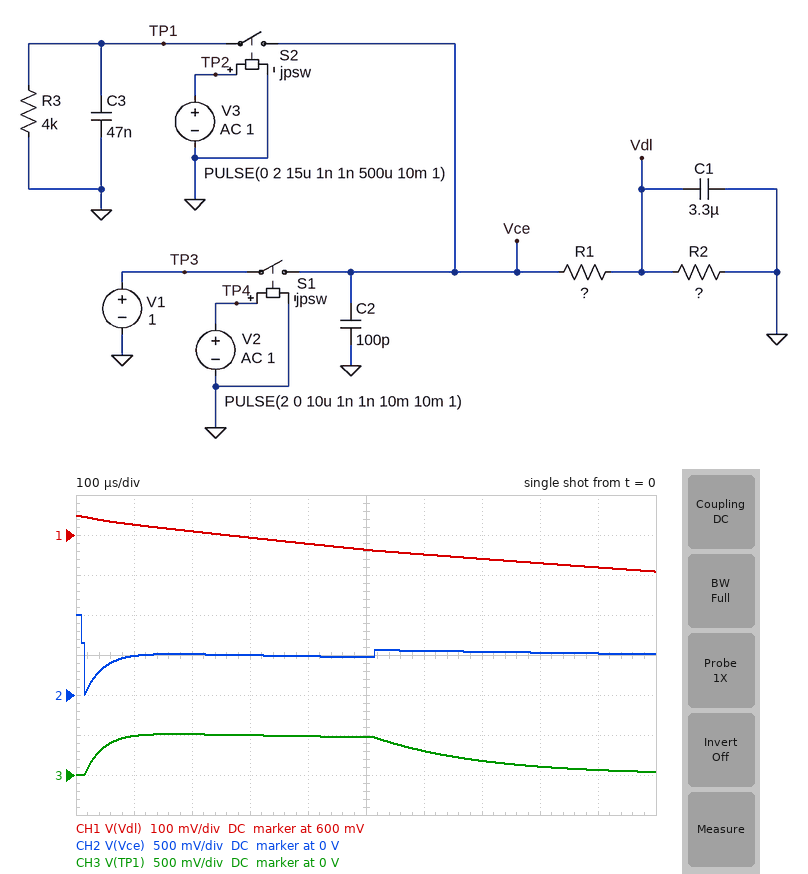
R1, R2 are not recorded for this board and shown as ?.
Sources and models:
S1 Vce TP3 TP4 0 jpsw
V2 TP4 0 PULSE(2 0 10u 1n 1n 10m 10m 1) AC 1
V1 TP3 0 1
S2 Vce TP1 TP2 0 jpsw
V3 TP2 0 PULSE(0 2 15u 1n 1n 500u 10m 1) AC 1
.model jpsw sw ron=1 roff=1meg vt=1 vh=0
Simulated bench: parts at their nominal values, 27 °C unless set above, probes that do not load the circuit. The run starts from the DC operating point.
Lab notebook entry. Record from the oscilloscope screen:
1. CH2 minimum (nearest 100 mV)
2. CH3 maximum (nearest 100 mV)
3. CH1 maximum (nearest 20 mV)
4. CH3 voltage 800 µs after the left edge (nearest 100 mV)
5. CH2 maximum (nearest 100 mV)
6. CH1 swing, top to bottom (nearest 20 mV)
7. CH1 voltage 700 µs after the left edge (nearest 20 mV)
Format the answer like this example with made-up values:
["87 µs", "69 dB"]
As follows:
["0 V", "500 mV", "640 mV", "100 mV", "1.0 V", "140 mV", "540 mV"]
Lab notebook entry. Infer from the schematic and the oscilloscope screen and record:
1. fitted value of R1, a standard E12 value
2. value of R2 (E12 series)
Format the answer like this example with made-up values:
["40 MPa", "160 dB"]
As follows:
["820 Ω", "1.5 kΩ"]
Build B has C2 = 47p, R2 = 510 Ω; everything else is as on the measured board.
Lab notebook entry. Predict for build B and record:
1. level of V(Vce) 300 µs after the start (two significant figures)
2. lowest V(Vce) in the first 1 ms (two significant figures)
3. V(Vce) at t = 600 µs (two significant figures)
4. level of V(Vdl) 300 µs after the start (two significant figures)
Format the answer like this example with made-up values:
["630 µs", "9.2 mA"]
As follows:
["270 mV", "4.8 mV", "260 mV", "310 mV"]
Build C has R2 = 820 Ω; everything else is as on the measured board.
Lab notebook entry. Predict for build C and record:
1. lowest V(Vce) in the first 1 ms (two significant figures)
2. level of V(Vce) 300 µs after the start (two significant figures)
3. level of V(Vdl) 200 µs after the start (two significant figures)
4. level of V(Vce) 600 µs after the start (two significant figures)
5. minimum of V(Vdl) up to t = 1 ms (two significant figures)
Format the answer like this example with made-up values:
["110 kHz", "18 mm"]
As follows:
["5.6 mV", "370 mV", "460 mV", "390 mV", "330 mV"]
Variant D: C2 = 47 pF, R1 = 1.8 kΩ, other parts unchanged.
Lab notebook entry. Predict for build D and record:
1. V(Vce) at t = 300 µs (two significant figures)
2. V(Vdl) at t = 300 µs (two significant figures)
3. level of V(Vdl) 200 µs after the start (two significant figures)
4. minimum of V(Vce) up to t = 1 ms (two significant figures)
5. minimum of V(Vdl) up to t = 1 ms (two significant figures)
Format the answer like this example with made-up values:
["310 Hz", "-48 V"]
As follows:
["290 mV", "420 mV", "430 mV", "4.6 mV", "360 mV"]
